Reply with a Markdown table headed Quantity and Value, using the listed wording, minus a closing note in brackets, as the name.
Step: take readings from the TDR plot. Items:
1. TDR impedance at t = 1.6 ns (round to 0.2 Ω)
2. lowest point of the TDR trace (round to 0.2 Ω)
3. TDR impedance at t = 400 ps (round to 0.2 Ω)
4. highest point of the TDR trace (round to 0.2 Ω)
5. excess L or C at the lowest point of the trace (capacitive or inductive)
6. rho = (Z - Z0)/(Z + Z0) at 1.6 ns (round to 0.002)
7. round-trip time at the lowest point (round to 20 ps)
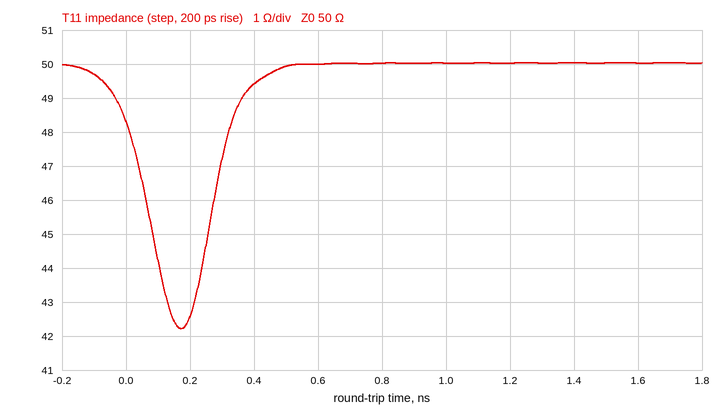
| Quantity | Value |
|---|---|
| TDR impedance at t = 1.6 ns | 50.0 Ω |
| lowest point of the TDR trace | 42.2 Ω |
| TDR impedance at t = 400 ps | 49.4 Ω |
| highest point of the TDR trace | 50.0 Ω |
| excess L or C at the lowest point of the trace | capacitive |
| rho = (Z - Z0)/(Z + Z0) at 1.6 ns | 0.000 |
| round-trip time at the lowest point | 180 ps |
